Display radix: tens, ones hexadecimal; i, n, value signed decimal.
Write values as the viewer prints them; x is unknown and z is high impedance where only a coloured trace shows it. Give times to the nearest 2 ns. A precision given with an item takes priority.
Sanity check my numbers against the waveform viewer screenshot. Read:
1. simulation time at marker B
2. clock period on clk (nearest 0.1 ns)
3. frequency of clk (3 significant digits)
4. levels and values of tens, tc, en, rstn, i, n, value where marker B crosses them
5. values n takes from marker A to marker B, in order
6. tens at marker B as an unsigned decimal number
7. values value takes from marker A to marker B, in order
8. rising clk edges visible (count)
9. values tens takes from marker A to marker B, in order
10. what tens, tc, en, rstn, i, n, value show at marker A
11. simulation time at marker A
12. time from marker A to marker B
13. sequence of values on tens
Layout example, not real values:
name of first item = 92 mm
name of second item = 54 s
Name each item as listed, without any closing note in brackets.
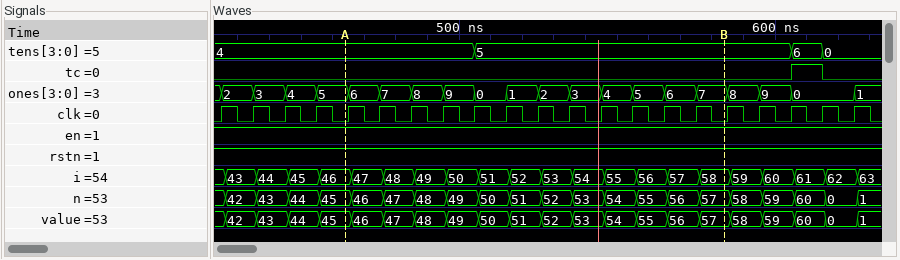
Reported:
simulation time at marker B = 584 ns
clock period on clk = 10 ns
frequency of clk = 100 MHz
levels and values of tens, tc, en, rstn, i, n, value where marker B crosses them = tens=5, tc=0, en=1, rstn=1, i=58, n=57, value=57
values n takes from marker A to marker B, in order = 45, 46, 47, 48, 49, 50, 51, 52, 53, 54, 55, 56, 57
tens at marker B as an unsigned decimal number = 5
values value takes from marker A to marker B, in order = 45, 46, 47, 48, 49, 50, 51, 52, 53, 54, 55, 56, 57
rising clk edges visible = 21
values tens takes from marker A to marker B, in order = 4, 5
what tens, tc, en, rstn, i, n, value show at marker A = tens=4, tc=0, en=1, rstn=1, i=46, n=45, value=45
simulation time at marker A = 464 ns
time from marker A to marker B = 120 ns
sequence of values on tens = 4, 5, 6, 0
